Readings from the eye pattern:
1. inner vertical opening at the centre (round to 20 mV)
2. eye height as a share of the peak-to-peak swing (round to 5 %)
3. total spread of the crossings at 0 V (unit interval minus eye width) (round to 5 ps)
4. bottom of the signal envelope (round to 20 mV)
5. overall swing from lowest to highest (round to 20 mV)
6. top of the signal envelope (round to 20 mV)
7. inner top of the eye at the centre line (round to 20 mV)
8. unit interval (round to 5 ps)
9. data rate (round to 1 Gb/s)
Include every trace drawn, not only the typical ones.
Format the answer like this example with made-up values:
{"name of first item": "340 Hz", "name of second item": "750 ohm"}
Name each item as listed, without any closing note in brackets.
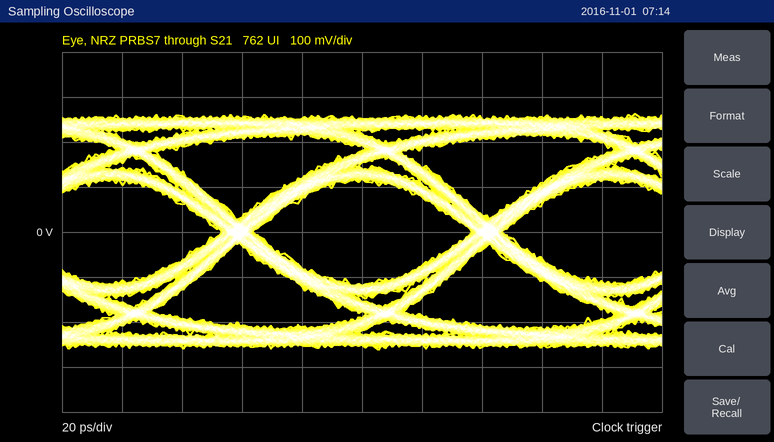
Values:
{"inner vertical opening at the centre": "240 mV", "eye height as a share of the peak-to-peak swing": "45 %", "total spread of the crossings at 0 V (unit interval minus eye width)": "10 ps", "bottom of the signal envelope": "-260 mV", "overall swing from lowest to highest": "520 mV", "top of the signal envelope": "260 mV", "inner top of the eye at the centre line": "120 mV", "unit interval": "85 ps", "data rate": "12 Gb/s"}
